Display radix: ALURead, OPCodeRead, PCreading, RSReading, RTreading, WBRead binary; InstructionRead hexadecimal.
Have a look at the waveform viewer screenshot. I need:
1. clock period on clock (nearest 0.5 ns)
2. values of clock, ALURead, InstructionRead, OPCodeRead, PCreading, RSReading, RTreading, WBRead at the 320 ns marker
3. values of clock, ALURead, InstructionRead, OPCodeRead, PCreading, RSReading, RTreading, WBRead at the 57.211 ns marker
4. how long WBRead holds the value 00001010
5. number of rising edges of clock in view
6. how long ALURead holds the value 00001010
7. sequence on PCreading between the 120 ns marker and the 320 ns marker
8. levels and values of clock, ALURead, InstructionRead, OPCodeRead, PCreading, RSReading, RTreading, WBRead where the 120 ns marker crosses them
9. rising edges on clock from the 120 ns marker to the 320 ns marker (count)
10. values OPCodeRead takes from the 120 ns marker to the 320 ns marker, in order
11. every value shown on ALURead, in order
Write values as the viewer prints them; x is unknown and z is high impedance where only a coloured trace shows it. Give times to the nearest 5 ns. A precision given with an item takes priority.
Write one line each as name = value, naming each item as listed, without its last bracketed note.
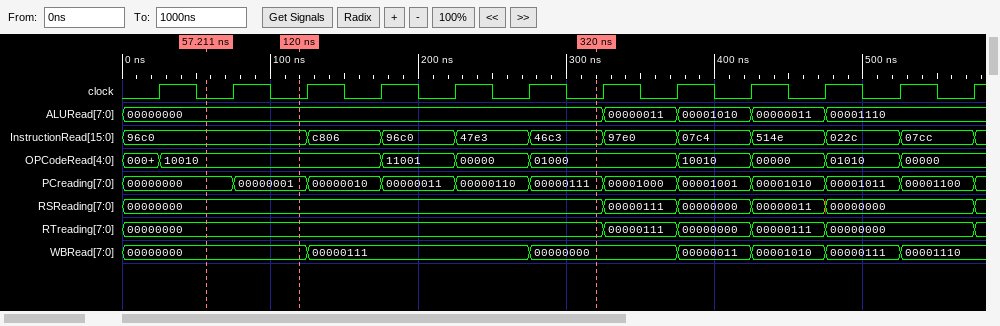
clock period on clock = 50 ns
values of clock, ALURead, InstructionRead, OPCodeRead, PCreading, RSReading, RTreading, WBRead at the 320 ns marker = clock=0, ALURead=00000000, InstructionRead=46c3, OPCodeRead=01000, PCreading=00000111, RSReading=00000000, RTreading=00000000, WBRead=00000000
values of clock, ALURead, InstructionRead, OPCodeRead, PCreading, RSReading, RTreading, WBRead at the 57.211 ns marker = clock=0, ALURead=00000000, InstructionRead=96c0, OPCodeRead=10010, PCreading=00000000, RSReading=00000000, RTreading=00000000, WBRead=00000000
how long WBRead holds the value 00001010 = 50 ns
number of rising edges of clock in view = 12
how long ALURead holds the value 00001010 = 50 ns
sequence on PCreading between the 120 ns marker and the 320 ns marker = 00000001, 00000010, 00000011, 00000110, 00000111
levels and values of clock, ALURead, InstructionRead, OPCodeRead, PCreading, RSReading, RTreading, WBRead where the 120 ns marker crosses them = clock=0, ALURead=00000000, InstructionRead=96c0, OPCodeRead=10010, PCreading=00000001, RSReading=00000000, RTreading=00000000, WBRead=00000000
rising edges on clock from the 120 ns marker to the 320 ns marker = 4
values OPCodeRead takes from the 120 ns marker to the 320 ns marker, in order = 10010, 11001, 00000, 01000
every value shown on ALURead, in order = 00000000, 00000011, 00001010, 00000011, 00001110
